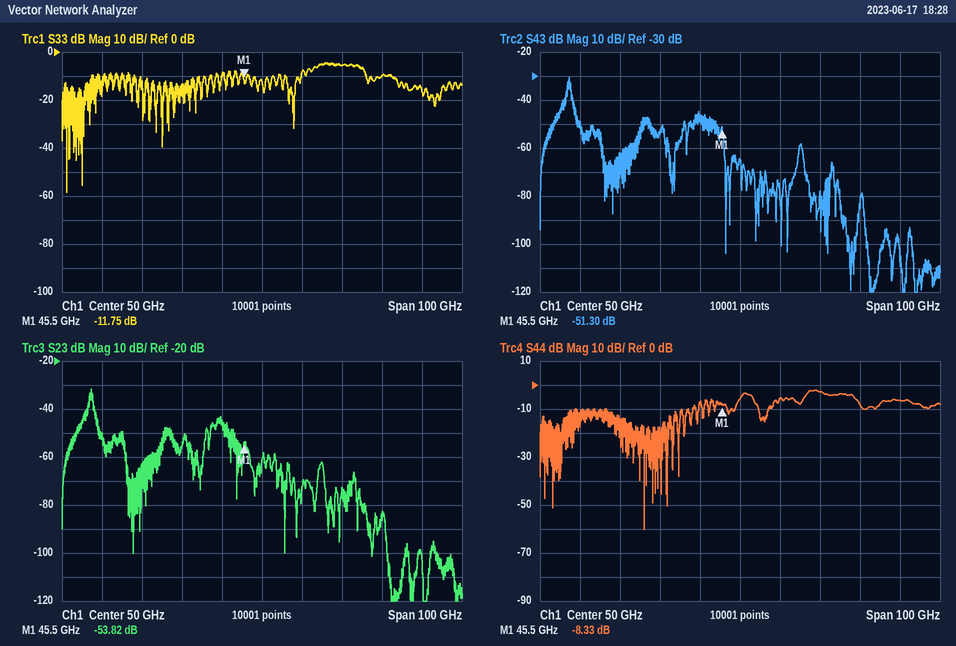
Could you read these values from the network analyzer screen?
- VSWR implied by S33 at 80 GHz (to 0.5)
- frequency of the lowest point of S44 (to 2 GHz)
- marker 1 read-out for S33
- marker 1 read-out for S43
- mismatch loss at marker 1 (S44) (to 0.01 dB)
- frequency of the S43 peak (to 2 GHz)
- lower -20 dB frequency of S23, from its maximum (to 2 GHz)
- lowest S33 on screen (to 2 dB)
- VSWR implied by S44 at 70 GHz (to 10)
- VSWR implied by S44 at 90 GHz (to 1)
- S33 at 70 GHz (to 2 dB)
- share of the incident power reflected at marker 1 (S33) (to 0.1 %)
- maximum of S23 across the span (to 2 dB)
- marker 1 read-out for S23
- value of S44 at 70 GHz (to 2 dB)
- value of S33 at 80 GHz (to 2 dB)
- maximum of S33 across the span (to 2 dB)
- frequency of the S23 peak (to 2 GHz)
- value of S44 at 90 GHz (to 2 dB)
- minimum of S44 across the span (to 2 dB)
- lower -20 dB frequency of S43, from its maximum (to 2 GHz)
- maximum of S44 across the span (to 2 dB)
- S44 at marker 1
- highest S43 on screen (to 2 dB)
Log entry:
2.0
26 GHz
-11.75 dB
-51.30 dB
0.69 dB
8 GHz
4 GHz
-58 dB
10
3
-6 dB
6.7 %
-32 dB
-53.82 dB
-2 dB
-10 dB
-4 dB
8 GHz
-6 dB
-60 dB
4 GHz
-2 dB
-8.33 dB
-30 dB
